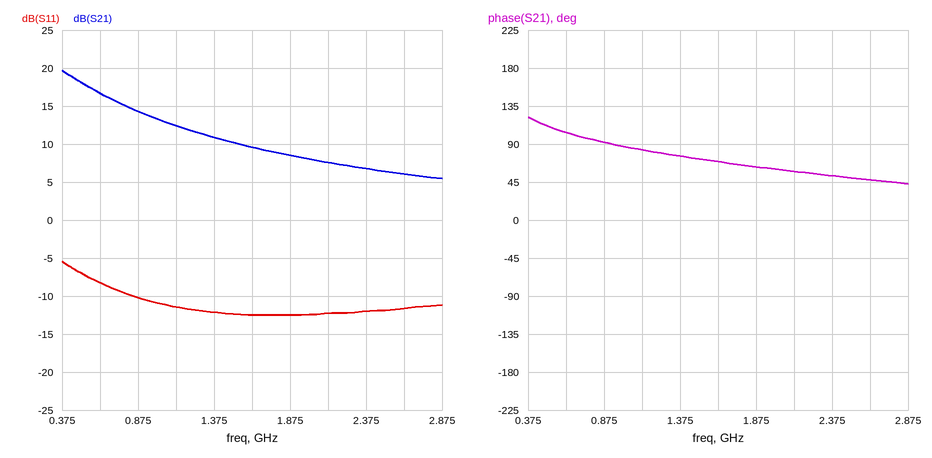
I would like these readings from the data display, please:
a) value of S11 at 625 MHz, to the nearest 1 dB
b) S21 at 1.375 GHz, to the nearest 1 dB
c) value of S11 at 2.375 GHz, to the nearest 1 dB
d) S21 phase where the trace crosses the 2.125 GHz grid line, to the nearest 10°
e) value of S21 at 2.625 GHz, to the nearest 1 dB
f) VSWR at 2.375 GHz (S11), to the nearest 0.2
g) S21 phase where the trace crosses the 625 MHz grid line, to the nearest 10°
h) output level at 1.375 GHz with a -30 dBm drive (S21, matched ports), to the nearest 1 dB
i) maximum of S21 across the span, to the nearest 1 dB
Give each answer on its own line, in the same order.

-8 dB
11 dB
-12 dB
60°
6 dB
1.6
100°
-19 dBm
20 dB
